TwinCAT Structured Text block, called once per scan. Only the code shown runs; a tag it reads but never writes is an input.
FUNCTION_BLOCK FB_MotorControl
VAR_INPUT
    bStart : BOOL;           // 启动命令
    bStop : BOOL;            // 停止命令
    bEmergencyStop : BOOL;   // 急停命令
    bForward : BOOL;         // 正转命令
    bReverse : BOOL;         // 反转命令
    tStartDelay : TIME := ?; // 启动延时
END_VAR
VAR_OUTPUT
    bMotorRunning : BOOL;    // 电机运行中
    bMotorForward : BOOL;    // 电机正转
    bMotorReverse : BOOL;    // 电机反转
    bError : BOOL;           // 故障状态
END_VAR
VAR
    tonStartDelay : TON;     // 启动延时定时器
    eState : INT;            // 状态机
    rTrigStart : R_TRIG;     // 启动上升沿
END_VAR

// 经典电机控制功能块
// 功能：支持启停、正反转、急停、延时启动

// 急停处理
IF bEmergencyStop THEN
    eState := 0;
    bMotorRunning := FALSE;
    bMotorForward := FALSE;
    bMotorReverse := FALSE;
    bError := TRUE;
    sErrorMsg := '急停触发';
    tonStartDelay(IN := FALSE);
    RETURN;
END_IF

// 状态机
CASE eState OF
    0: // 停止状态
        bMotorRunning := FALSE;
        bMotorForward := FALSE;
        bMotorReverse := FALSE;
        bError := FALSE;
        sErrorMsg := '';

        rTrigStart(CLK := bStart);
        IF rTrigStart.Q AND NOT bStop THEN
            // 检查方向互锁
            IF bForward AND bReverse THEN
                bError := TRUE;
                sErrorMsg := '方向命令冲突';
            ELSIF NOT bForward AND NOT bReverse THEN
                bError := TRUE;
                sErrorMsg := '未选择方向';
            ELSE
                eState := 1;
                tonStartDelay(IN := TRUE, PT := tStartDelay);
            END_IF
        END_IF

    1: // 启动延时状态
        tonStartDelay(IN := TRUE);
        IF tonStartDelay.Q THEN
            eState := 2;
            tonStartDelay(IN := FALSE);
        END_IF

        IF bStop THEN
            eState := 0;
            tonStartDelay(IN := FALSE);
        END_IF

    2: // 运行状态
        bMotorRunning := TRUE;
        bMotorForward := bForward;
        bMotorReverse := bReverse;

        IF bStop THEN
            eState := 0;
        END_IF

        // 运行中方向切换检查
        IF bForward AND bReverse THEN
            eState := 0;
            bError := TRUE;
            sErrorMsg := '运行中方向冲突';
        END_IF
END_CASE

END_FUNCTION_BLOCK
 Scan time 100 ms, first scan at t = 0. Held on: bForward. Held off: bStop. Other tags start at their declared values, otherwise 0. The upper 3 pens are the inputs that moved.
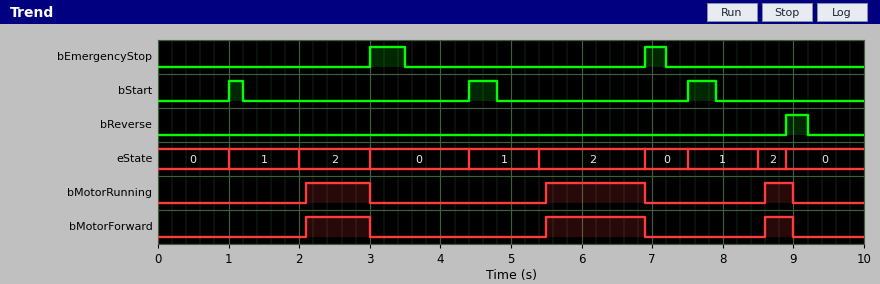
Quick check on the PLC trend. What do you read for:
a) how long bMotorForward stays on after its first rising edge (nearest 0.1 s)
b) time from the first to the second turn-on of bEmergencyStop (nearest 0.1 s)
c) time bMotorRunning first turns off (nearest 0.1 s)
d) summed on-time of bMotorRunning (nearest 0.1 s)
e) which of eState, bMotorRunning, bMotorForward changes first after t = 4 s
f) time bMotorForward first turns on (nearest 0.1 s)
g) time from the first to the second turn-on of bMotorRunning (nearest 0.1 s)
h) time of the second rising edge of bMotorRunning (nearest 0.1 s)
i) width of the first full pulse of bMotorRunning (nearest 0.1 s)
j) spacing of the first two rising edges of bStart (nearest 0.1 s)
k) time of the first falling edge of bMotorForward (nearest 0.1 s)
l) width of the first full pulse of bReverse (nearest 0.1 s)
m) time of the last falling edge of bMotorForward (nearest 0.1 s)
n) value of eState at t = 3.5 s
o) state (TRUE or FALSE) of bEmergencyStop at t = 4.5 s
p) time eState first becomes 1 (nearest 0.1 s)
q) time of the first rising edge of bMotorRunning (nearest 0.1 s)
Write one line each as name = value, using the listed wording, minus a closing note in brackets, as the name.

how long bMotorForward stays on after its first rising edge = 0.9 s
time from the first to the second turn-on of bEmergencyStop = 3.9 s
time bMotorRunning first turns off = 3.0 s
summed on-time of bMotorRunning = 2.7 s
which of eState, bMotorRunning, bMotorForward changes first after t = 4 s = eState
time bMotorForward first turns on = 2.1 s
time from the first to the second turn-on of bMotorRunning = 3.4 s
time of the second rising edge of bMotorRunning = 5.5 s
width of the first full pulse of bMotorRunning = 0.9 s
spacing of the first two rising edges of bStart = 3.4 s
time of the first falling edge of bMotorForward = 3.0 s
width of the first full pulse of bReverse = 0.3 s
time of the last falling edge of bMotorForward = 9.0 s
value of eState at t = 3.5 s = 0
state (TRUE or FALSE) of bEmergencyStop at t = 4.5 s = FALSE
time eState first becomes 1 = 1.0 s
time of the first rising edge of bMotorRunning = 2.1 s
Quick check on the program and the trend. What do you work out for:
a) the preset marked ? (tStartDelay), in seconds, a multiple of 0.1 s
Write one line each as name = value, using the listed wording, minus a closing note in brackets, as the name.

the preset marked ? (tStartDelay), in seconds, a multiple of 0.1 s = 1.0 s
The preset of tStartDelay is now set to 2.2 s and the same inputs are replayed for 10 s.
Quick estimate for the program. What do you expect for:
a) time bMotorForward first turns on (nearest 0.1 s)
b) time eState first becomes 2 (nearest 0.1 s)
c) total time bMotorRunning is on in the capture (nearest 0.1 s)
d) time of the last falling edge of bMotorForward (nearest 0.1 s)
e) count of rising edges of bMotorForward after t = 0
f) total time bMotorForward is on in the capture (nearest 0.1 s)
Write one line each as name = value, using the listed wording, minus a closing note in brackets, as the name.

time bMotorForward first turns on = 6.7 s
time eState first becomes 2 = 6.6 s
total time bMotorRunning is on in the capture = 0.4 s
time of the last falling edge of bMotorForward = 6.9 s
count of rising edges of bMotorForward after t = 0 = 2
total time bMotorForward is on in the capture = 0.4 s
